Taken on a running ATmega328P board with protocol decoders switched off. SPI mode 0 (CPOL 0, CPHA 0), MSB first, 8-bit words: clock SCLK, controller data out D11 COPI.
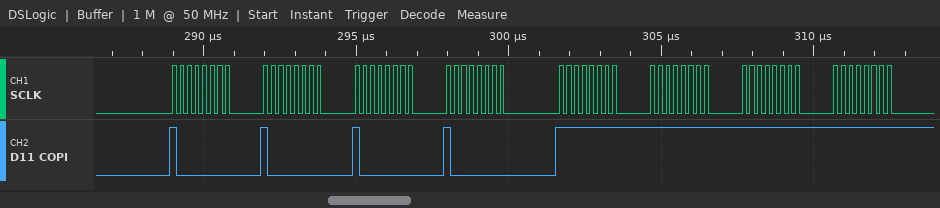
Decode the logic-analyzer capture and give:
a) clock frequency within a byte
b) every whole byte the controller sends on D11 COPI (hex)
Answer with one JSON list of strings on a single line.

["4 MHz", "80 80 80 80 FF FF FF FF"]
